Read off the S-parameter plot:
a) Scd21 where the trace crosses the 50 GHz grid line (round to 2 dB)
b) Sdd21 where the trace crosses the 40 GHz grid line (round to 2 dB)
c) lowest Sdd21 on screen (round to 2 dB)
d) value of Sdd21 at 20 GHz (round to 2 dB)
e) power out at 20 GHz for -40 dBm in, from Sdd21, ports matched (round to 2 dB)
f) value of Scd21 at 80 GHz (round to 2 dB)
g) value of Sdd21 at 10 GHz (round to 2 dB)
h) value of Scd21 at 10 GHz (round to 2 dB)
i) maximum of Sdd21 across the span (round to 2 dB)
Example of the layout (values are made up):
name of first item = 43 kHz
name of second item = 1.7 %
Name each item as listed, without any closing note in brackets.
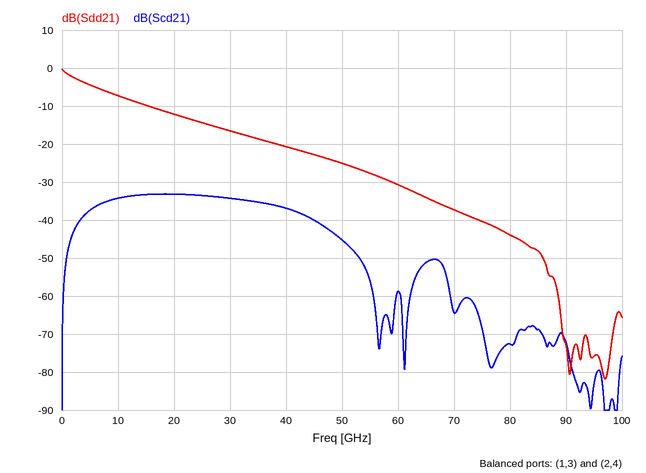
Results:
Scd21 where the trace crosses the 50 GHz grid line = -46 dB
Sdd21 where the trace crosses the 40 GHz grid line = -20 dB
lowest Sdd21 on screen = -82 dB
value of Sdd21 at 20 GHz = -12 dB
power out at 20 GHz for -40 dBm in, from Sdd21, ports matched = -52 dBm
value of Scd21 at 80 GHz = -72 dB
value of Sdd21 at 10 GHz = -8 dB
value of Scd21 at 10 GHz = -34 dB
maximum of Sdd21 across the span = 0 dB
